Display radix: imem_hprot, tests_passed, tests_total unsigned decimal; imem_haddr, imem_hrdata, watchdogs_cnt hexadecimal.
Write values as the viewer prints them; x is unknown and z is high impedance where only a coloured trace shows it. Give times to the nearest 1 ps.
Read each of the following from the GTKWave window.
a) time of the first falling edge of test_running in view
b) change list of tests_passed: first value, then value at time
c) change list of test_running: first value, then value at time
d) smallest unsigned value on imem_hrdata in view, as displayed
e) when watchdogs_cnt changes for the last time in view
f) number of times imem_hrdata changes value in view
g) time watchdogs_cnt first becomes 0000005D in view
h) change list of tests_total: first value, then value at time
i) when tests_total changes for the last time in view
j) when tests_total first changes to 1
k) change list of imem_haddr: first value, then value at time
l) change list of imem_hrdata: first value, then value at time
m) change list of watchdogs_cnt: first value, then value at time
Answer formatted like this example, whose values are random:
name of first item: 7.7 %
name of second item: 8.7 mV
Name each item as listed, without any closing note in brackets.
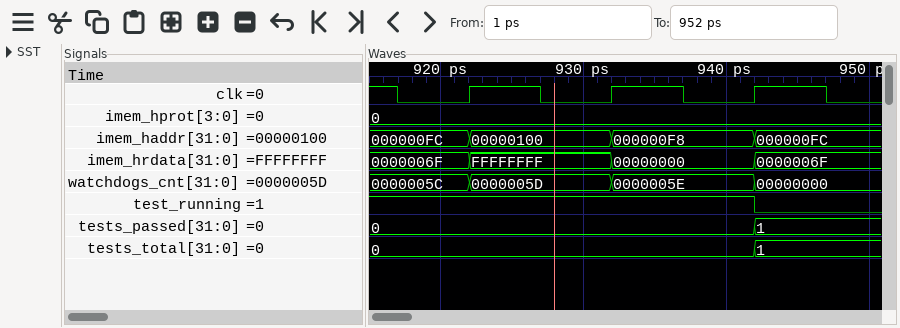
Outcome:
time of the first falling edge of test_running in view: 942 ps
change list of tests_passed: first value, then value at time: 0, 1 at 942 ps
change list of test_running: first value, then value at time: 1, 0 at 942 ps
smallest unsigned value on imem_hrdata in view, as displayed: 00000000
when watchdogs_cnt changes for the last time in view: 942 ps
number of times imem_hrdata changes value in view: 3
time watchdogs_cnt first becomes 0000005D in view: 922 ps
change list of tests_total: first value, then value at time: 0, 1 at 942 ps
when tests_total changes for the last time in view: 942 ps
when tests_total first changes to 1: 942 ps
change list of imem_haddr: first value, then value at time: 000000FC, 00000100 at 922 ps, 000000F8 at 932 ps, 000000FC at 942 ps
change list of imem_hrdata: first value, then value at time: 0000006F, FFFFFFFF at 922 ps, 00000000 at 932 ps, 0000006F at 942 ps
change list of watchdogs_cnt: first value, then value at time: 0000005C, 0000005D at 922 ps, 0000005E at 932 ps, 00000000 at 942 ps
